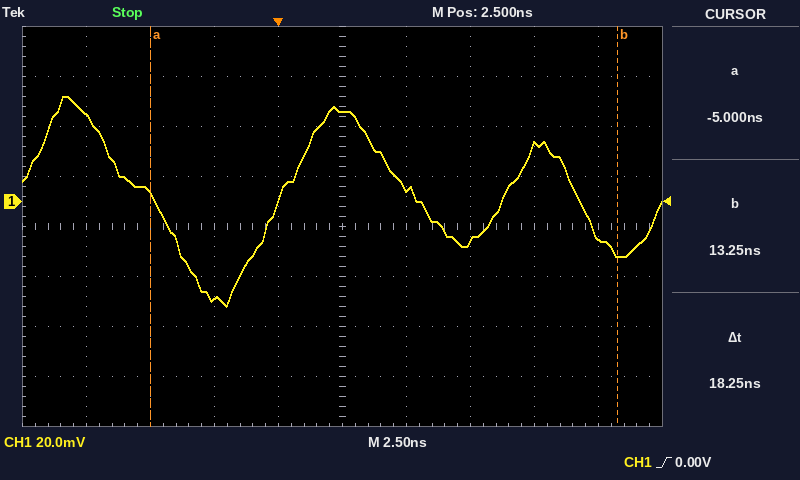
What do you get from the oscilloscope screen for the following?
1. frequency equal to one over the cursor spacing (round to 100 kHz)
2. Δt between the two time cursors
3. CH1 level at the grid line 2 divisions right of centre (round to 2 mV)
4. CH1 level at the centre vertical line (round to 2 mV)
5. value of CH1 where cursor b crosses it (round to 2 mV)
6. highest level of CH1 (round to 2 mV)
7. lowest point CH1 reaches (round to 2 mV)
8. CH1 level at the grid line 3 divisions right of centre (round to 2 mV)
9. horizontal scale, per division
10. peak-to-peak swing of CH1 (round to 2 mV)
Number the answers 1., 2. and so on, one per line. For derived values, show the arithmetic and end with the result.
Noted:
1. 1 / 18.25 ns ≈ 54.8 MHz
2. 18.25 ns
3. -16 mV
4. 36 mV
5. -22 mV
6. 42 mV
7. -42 mV
8. 22 mV
9. 2.5 ns
10. 42 mV − (-42 mV) = 84 mV
